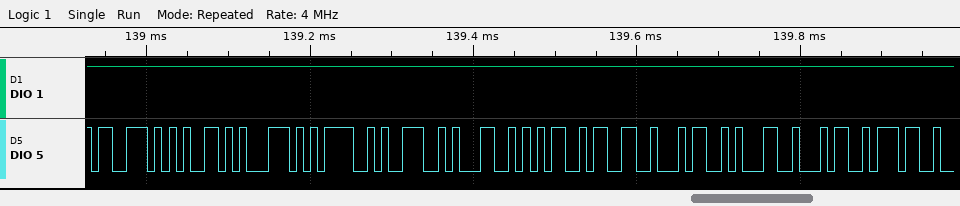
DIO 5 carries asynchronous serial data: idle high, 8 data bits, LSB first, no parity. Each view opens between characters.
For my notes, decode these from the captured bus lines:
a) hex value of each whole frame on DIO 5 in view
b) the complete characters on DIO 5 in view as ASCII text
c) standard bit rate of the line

73, 65, 71, 3D, 39, 31, 35, 33, 34, 31, 34, 37
"seq=91534147"
115200 baud
